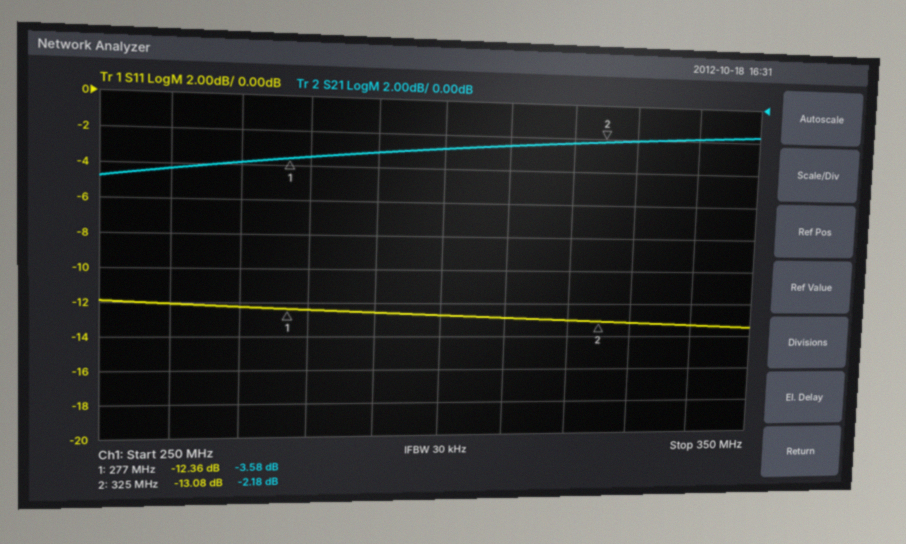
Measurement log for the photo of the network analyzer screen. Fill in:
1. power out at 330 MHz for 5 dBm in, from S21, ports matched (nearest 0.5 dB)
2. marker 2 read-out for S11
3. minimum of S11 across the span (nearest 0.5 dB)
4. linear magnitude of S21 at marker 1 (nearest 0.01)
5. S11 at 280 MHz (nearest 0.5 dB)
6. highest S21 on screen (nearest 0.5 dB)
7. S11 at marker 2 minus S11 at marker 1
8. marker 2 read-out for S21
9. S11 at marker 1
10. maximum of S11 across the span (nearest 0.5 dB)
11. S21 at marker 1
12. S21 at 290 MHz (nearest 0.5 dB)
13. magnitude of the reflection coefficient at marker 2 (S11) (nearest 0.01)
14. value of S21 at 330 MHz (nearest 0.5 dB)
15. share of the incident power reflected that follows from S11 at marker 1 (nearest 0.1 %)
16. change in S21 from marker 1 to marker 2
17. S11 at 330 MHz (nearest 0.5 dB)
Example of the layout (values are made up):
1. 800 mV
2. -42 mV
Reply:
1. 3.0 dBm
2. -13.08 dB
3. -13.5 dB
4. 0.66
5. -12.5 dB
6. -1.5 dB
7. -0.72 dB
8. -2.18 dB
9. -12.36 dB
10. -12.0 dB
11. -3.58 dB
12. -3.0 dB
13. 0.22
14. -2.0 dB
15. 5.8 %
16. 1.40 dB
17. -13.0 dB
